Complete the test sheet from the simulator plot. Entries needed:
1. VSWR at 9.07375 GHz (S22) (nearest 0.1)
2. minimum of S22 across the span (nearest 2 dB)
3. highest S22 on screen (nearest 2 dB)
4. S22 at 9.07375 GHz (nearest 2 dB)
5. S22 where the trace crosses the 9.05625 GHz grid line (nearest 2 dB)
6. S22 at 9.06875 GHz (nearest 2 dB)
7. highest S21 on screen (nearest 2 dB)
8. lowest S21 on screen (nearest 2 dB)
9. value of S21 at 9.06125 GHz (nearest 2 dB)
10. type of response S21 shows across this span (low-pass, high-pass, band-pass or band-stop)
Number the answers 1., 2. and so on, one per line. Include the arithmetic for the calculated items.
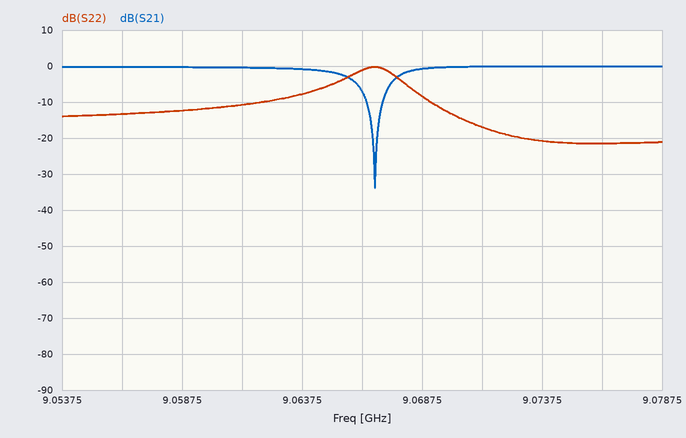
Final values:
1. |Γ| = 10^(-20/20) = 0.1000; VSWR = (1 + 0.1000)/(1 − 0.1000) ≈ 1.2
2. -22 dB
3. 0 dB
4. -20 dB
5. -14 dB
6. -8 dB
7. 0 dB
8. -34 dB
9. 0 dB
10. band-stop
